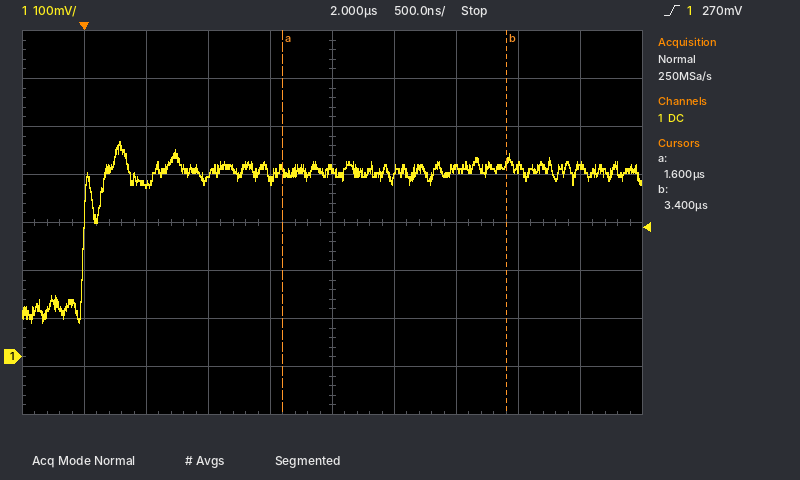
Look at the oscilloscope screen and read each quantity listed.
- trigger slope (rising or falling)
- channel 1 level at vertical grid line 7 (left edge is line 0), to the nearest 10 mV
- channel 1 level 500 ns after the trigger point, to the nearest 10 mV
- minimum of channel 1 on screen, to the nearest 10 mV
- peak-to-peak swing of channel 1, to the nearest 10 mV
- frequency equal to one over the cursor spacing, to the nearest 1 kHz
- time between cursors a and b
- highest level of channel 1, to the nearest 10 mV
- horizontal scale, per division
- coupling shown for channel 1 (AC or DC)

rising
390 mV
360 mV
70 mV
380 mV
556 kHz
1.80 µs
450 mV
500 ns
DC
